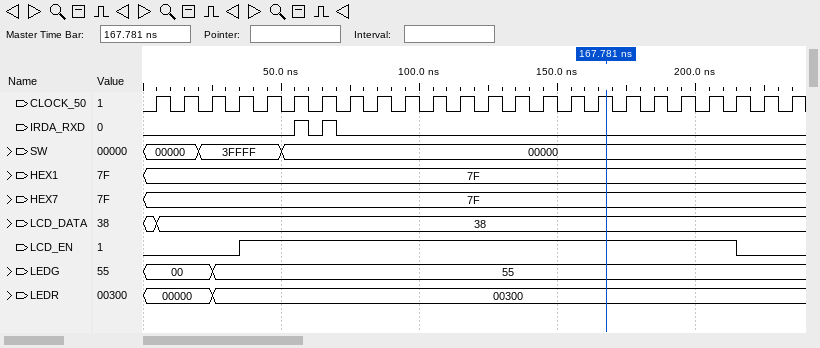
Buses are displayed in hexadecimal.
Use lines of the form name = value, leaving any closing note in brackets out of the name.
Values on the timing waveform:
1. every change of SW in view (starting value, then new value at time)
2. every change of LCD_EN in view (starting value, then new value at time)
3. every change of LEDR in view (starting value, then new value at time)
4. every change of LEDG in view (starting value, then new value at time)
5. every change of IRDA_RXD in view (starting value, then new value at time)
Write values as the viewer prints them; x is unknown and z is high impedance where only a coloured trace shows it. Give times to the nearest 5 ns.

every change of SW in view = 00000, 3FFFF at 20 ns, 00000 at 50 ns
every change of LCD_EN in view = 0, 1 at 35 ns, 0 at 215 ns
every change of LEDR in view = 00000, 00300 at 25 ns
every change of LEDG in view = 00, 55 at 25 ns
every change of IRDA_RXD in view = 0, 1 at 55 ns, 0 at 60 ns, 1 at 65 ns, 0 at 70 ns
